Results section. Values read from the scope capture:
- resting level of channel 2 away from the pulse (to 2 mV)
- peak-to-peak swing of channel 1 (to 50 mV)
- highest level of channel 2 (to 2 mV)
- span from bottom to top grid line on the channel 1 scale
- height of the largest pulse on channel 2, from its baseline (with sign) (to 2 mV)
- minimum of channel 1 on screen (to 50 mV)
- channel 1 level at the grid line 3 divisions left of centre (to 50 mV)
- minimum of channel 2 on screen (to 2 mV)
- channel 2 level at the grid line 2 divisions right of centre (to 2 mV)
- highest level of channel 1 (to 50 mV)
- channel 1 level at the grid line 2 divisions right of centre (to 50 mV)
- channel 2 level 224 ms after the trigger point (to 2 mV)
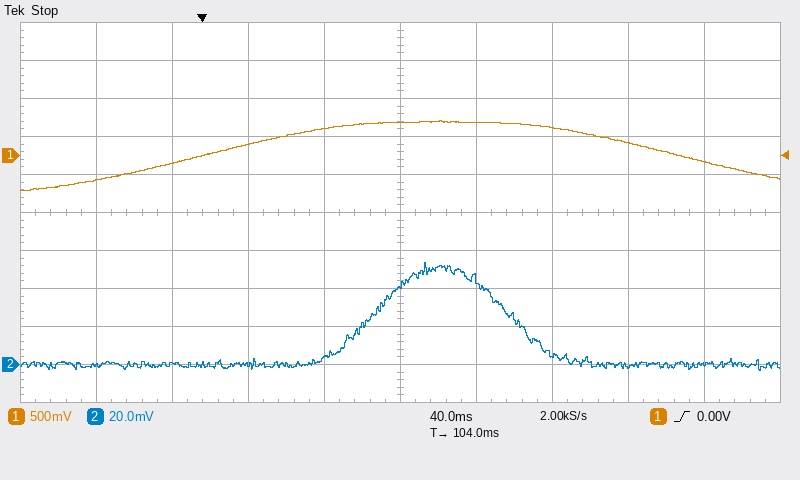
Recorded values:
0 mV
900 mV
54 mV
5 V
+54 mV
-450 mV
-100 mV
-4 mV
6 mV
450 mV
350 mV
0 mV
